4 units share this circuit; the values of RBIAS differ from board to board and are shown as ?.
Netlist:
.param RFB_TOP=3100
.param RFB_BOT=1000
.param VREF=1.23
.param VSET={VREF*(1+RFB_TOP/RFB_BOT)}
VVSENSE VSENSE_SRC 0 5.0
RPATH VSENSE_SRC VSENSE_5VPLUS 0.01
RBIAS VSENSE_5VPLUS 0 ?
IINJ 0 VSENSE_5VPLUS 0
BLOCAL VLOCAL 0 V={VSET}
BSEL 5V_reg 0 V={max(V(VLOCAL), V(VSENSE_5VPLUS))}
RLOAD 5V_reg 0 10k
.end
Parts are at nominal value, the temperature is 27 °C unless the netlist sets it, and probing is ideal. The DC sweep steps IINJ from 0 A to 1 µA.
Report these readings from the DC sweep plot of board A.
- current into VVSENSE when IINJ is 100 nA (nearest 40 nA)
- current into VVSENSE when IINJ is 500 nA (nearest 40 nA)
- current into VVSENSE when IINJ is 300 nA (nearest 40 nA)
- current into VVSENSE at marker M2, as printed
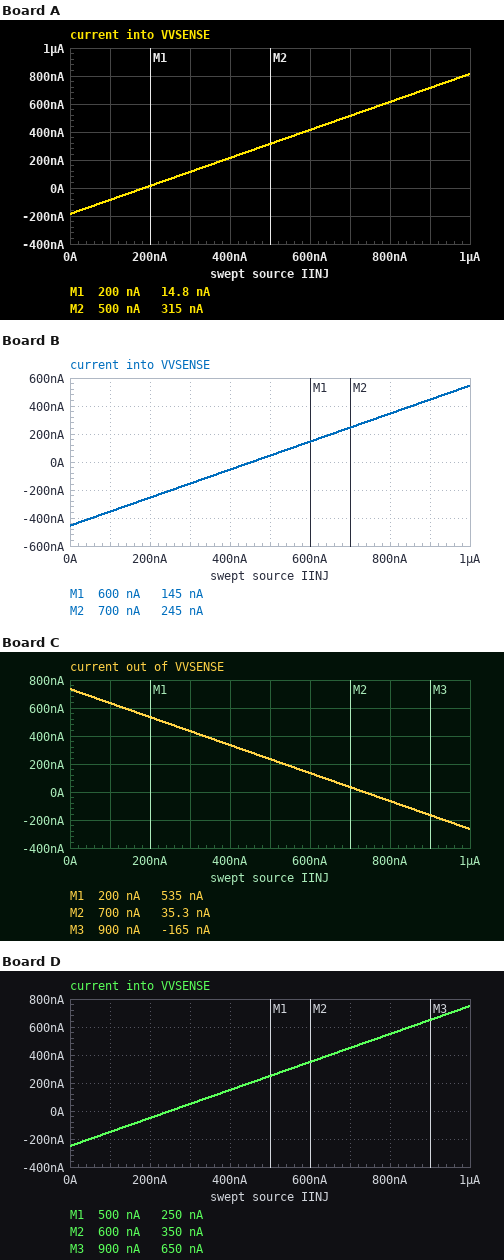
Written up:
-80 nA
320 nA
120 nA
315 nA
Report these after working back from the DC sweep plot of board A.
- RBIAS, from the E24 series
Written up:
27 MΩ
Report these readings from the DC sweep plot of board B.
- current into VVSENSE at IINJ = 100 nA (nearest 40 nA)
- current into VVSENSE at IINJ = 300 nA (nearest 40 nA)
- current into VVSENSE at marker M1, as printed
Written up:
-360 nA
-160 nA
145 nA
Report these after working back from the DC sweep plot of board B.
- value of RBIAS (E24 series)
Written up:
11 MΩ
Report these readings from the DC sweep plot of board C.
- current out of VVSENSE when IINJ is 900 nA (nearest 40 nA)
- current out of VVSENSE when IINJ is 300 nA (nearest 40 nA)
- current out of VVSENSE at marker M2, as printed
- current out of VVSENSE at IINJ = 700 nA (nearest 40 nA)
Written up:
-160 nA
440 nA
35.3 nA
40 nA
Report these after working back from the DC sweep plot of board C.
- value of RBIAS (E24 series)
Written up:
6.8 MΩ
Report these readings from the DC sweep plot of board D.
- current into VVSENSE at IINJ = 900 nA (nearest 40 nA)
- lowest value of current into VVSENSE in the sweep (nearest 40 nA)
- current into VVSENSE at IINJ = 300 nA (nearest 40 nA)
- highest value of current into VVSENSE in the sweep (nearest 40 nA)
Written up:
640 nA
-240 nA
40 nA
760 nA
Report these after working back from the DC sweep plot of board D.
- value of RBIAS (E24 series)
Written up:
20 MΩ
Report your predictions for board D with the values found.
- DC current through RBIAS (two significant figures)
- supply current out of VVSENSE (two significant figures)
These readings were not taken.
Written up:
250 nA
250 nA
